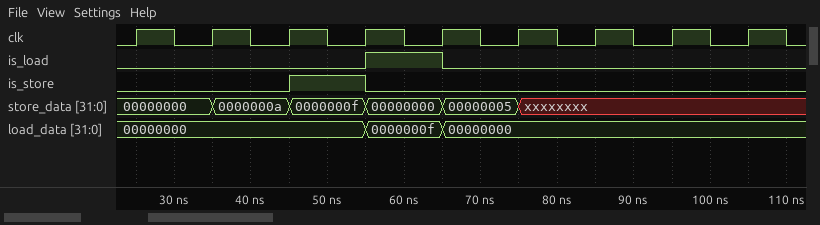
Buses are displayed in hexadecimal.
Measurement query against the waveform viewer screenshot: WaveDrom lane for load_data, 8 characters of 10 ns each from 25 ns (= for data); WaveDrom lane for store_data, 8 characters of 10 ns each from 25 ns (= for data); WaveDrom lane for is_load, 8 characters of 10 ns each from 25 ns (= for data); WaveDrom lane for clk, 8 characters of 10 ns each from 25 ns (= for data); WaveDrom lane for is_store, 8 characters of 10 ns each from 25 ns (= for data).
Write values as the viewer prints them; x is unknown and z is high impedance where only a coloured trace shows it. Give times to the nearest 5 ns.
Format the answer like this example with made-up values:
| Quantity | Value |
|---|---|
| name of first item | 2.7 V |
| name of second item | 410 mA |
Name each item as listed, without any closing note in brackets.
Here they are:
| Quantity | Value |
|---|---|
| WaveDrom lane for load_data, 8 characters of 10 ns each from 25 ns | {name: 'load_data', wave: '=..==...', data: '00000000 0000000f 00000000'} |
| WaveDrom lane for store_data, 8 characters of 10 ns each from 25 ns | {name: 'store_data', wave: '=====x..', data: '00000000 0000000a 0000000f 00000000 00000005'} |
| WaveDrom lane for is_load, 8 characters of 10 ns each from 25 ns | {name: 'is_load', wave: '0..10...'} |
| WaveDrom lane for clk, 8 characters of 10 ns each from 25 ns | {name: 'clk', wave: 'p.......'} |
| WaveDrom lane for is_store, 8 characters of 10 ns each from 25 ns | {name: 'is_store', wave: '0.10....'} |
